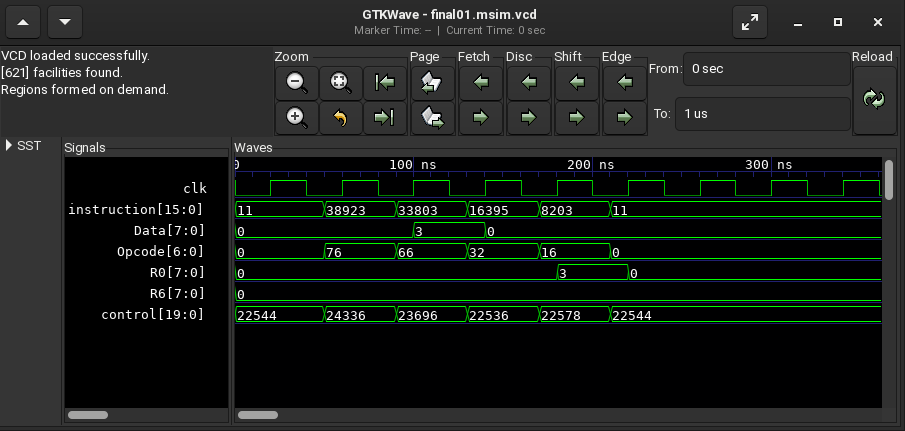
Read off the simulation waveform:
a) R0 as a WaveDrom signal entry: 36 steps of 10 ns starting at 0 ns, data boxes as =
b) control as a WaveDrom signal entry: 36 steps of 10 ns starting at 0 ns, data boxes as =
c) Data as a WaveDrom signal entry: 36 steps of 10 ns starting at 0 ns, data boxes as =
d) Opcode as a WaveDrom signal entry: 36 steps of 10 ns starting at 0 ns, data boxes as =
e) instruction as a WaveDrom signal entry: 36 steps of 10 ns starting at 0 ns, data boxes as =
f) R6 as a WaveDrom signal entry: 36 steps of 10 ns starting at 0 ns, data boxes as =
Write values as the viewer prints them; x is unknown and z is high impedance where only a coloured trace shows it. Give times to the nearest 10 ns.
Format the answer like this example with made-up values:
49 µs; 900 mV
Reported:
{name: 'R0', wave: '=.................=...=.............', data: '0 3 0'}; {name: 'control', wave: '=....=...=...=...=...=..............', data: '22544 24336 23696 22536 22578 22544'}; {name: 'Data', wave: '=.........=...=.....................', data: '0 3 0'}; {name: 'Opcode', wave: '=....=...=...=...=...=..............', data: '0 76 66 32 16 0'}; {name: 'instruction', wave: '=....=...=...=...=...=..............', data: '11 38923 33803 16395 8203 11'}; {name: 'R6', wave: '=...................................', data: '0'}
